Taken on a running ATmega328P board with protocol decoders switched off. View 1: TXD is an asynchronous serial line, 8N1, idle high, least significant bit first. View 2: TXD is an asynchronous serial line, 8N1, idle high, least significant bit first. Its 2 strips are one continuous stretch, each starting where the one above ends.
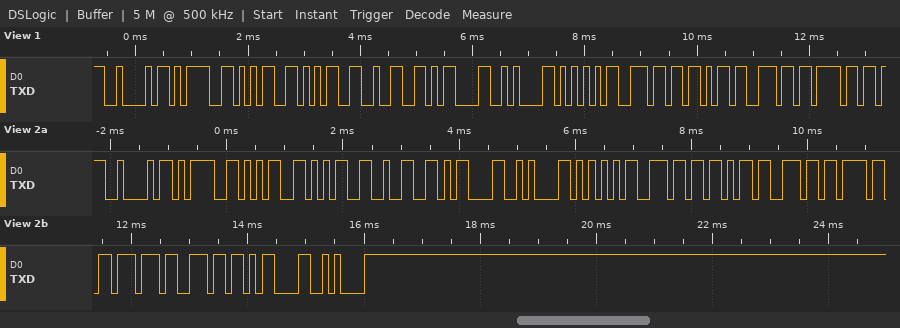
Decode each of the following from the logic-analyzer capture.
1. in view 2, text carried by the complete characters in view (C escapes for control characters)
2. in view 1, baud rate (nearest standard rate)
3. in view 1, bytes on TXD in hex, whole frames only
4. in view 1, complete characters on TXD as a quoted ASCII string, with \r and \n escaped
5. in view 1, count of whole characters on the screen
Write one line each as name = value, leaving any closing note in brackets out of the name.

in view 2, text carried by the complete characters in view = "B=552\r\nUnknown\r\n"
in view 1, baud rate = 9600 baud
in view 1, bytes on TXD in hex, whole frames only = 0x42 0x3D 0x35 0x35 0x32 0x0D 0x0A 0x55 0x6E 0x6B 0x6E 0x6F
in view 1, complete characters on TXD as a quoted ASCII string, with \r and \n escaped = "B=552\r\nUnkno"
in view 1, count of whole characters on the screen = 12
